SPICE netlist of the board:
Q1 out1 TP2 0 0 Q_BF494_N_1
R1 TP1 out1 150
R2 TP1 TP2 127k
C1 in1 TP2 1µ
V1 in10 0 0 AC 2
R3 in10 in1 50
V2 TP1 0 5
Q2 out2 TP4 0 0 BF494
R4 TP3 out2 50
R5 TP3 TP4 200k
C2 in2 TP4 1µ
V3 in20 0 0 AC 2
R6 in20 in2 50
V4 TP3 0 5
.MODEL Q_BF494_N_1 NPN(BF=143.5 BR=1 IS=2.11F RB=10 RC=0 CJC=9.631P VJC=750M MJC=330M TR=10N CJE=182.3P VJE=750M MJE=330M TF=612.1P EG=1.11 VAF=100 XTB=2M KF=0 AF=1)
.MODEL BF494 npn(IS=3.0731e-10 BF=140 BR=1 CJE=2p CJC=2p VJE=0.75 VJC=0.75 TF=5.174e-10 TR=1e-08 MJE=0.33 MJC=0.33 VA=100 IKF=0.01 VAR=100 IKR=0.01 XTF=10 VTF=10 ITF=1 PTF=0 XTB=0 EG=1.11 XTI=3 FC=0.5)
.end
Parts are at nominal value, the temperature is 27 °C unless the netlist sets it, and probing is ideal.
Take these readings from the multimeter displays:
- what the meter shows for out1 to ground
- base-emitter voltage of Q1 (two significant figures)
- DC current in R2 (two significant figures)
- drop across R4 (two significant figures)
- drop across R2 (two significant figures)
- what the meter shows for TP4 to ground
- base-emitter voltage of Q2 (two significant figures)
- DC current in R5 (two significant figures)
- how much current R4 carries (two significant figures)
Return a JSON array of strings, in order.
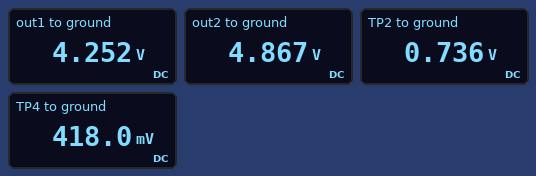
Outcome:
["4.252 V", "740 mV", "34 µA", "130 mV", "4.3 V", "418.0 mV", "420 mV", "23 µA", "2.7 mA"]
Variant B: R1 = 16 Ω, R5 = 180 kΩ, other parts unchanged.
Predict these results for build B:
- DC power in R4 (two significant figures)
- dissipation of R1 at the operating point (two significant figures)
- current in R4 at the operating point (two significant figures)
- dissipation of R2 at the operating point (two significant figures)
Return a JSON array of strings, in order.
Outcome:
["420 µW", "400 µW", "2.9 mA", "140 µW"]
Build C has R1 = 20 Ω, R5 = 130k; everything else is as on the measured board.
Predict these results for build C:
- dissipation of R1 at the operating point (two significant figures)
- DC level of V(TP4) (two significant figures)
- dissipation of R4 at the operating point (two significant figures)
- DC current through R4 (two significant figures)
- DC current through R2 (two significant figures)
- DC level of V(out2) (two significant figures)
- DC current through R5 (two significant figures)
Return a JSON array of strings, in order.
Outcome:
["500 µW", "430 mV", "710 µW", "3.8 mA", "34 µA", "4.8 V", "35 µA"]
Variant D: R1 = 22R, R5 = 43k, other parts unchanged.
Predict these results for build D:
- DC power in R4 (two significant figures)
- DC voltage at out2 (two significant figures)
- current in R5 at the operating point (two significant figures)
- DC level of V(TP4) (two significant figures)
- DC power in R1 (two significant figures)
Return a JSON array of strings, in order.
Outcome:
["3.6 mW", "4.6 V", "110 µA", "460 mV", "550 µW"]
